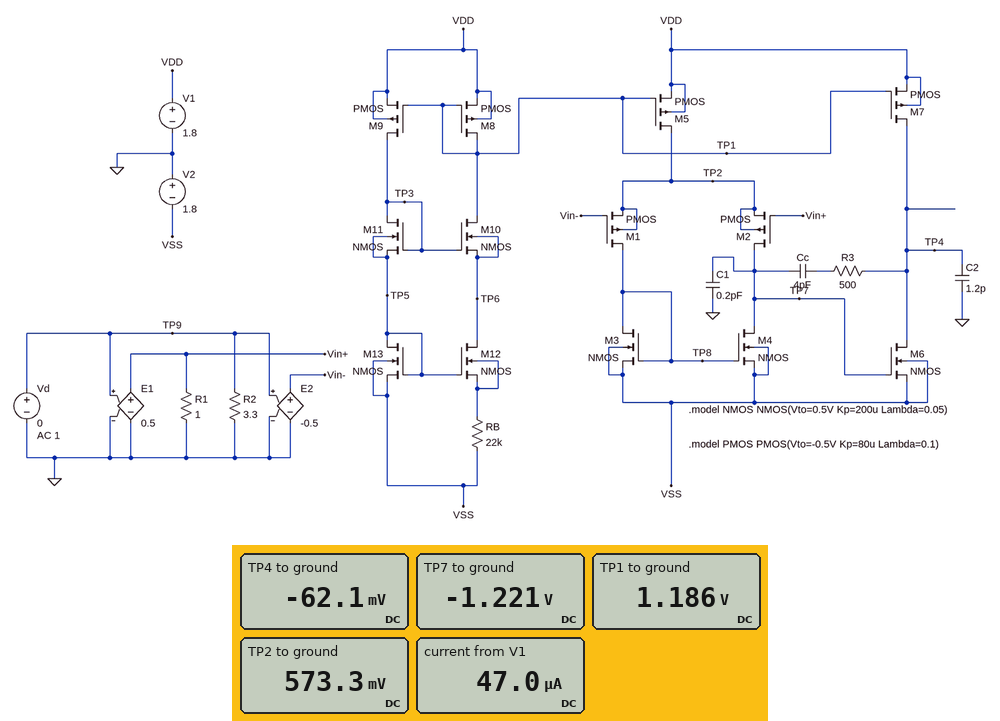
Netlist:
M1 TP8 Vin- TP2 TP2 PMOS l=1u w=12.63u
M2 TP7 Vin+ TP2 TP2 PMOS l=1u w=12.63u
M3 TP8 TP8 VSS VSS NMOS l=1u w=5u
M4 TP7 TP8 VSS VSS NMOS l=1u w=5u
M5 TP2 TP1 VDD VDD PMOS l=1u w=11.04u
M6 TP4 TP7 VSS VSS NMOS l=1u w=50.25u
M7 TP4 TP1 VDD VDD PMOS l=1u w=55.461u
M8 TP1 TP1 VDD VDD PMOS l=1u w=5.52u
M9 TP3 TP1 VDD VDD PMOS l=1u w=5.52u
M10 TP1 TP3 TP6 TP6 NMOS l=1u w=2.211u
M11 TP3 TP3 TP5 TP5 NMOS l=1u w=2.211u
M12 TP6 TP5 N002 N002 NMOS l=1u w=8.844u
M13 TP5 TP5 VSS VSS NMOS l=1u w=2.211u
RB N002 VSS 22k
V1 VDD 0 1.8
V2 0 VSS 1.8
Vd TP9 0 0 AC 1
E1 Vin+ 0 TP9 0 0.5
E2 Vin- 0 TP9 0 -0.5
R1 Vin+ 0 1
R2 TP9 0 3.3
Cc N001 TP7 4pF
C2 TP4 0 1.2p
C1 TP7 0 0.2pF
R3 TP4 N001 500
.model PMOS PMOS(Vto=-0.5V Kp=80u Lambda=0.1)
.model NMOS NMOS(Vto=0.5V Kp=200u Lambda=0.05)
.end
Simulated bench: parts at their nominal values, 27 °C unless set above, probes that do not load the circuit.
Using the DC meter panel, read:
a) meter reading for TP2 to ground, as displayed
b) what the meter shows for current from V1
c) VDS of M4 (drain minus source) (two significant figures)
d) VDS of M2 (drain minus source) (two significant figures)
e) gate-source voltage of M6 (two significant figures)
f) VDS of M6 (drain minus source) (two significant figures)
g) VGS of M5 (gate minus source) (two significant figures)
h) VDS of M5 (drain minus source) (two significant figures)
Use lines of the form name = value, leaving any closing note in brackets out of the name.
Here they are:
meter reading for TP2 to ground, as displayed = 573.3 mV
what the meter shows for current from V1 = 47.0 µA
VDS of M4 (drain minus source) = 580 mV
VDS of M2 (drain minus source) = -1.8 V
gate-source voltage of M6 = 580 mV
VDS of M6 (drain minus source) = 1.7 V
VGS of M5 (gate minus source) = -610 mV
VDS of M5 (drain minus source) = -1.2 V
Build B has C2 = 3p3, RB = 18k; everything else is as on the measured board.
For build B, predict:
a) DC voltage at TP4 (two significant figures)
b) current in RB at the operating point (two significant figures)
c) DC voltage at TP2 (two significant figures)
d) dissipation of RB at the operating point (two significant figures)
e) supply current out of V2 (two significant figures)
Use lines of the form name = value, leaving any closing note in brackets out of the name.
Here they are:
DC voltage at TP4 = -45 mV
current in RB at the operating point = 4.5 µA
DC voltage at TP2 = 590 mV
dissipation of RB at the operating point = 360 nW
supply current out of V2 = 69 µA
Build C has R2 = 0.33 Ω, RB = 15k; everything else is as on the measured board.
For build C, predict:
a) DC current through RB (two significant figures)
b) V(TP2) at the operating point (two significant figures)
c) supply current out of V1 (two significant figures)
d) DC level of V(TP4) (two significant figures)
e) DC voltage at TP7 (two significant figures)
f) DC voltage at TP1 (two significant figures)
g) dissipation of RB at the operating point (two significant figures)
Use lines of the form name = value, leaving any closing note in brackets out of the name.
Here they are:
DC current through RB = 6.3 µA
V(TP2) at the operating point = 610 mV
supply current out of V1 = 97 µA
DC level of V(TP4) = -27 mV
DC voltage at TP7 = -1.2 V
DC voltage at TP1 = 1.1 V
dissipation of RB at the operating point = 600 nW
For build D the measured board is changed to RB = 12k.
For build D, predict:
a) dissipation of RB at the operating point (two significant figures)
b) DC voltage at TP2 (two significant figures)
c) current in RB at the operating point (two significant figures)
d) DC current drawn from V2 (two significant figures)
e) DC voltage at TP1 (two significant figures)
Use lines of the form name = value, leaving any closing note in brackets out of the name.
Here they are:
dissipation of RB at the operating point = 1.1 µW
DC voltage at TP2 = 630 mV
current in RB at the operating point = 9.7 µA
DC current drawn from V2 = 150 µA
DC voltage at TP1 = 1.1 V
